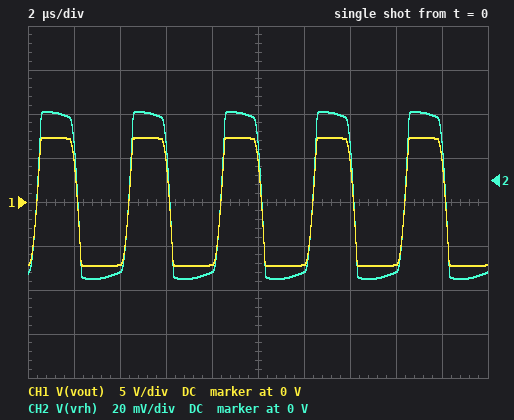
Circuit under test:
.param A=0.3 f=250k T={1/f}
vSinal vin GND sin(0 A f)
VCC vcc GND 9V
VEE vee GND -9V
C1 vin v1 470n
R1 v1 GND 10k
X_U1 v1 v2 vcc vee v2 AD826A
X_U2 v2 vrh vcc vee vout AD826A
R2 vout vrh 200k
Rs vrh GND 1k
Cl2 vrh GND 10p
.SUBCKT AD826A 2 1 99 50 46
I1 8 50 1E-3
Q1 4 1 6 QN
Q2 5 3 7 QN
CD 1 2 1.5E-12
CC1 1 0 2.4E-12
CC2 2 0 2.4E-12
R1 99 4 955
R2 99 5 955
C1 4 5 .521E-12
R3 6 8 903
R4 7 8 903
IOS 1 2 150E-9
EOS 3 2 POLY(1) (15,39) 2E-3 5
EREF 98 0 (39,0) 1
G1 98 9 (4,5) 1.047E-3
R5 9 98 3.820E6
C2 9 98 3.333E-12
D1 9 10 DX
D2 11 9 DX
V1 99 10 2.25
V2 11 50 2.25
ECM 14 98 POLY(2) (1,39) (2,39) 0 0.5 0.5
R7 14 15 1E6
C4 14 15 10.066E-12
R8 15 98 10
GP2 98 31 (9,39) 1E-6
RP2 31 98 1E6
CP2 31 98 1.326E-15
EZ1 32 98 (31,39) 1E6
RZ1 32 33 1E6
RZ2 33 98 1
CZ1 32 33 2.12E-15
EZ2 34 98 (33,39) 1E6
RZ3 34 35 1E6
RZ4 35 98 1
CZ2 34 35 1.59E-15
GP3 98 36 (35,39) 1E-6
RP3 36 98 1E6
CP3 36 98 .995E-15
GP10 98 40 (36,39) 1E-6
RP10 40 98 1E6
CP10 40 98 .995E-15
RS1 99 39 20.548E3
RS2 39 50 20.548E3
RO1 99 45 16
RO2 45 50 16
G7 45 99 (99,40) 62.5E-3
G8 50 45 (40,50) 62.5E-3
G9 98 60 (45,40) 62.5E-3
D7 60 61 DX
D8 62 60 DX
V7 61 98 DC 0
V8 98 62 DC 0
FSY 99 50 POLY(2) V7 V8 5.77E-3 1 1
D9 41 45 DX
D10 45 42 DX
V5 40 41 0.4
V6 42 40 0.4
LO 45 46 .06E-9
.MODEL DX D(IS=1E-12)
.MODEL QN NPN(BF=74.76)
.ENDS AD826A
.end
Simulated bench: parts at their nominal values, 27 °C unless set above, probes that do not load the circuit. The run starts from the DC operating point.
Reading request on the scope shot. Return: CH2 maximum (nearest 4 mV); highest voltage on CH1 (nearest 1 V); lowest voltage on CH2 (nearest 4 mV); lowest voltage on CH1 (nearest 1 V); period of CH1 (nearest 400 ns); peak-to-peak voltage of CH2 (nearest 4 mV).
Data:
32 mV
7 V
-44 mV
-7 V
4.0 µs
76 mV
